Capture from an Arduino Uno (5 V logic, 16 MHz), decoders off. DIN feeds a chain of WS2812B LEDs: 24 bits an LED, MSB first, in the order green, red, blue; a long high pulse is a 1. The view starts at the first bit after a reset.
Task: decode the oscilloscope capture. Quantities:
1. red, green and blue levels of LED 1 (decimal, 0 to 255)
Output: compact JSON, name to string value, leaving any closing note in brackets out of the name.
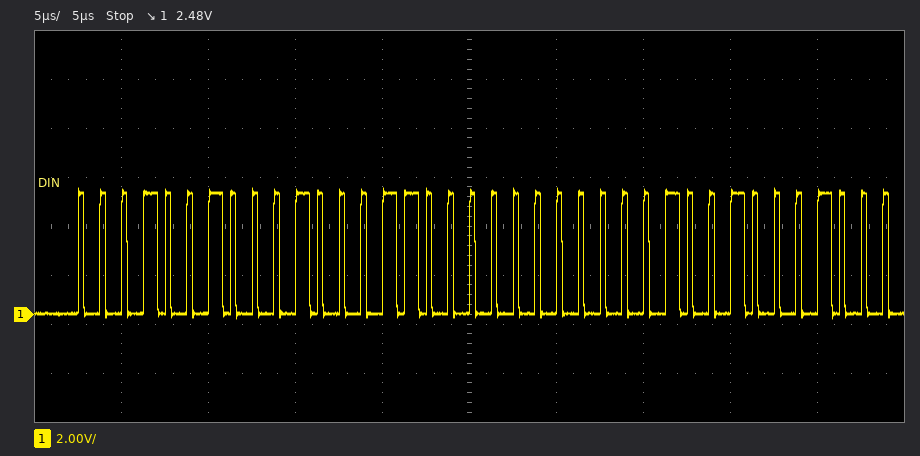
{"red, green and blue levels of LED 1": "35, 18, 0"}
